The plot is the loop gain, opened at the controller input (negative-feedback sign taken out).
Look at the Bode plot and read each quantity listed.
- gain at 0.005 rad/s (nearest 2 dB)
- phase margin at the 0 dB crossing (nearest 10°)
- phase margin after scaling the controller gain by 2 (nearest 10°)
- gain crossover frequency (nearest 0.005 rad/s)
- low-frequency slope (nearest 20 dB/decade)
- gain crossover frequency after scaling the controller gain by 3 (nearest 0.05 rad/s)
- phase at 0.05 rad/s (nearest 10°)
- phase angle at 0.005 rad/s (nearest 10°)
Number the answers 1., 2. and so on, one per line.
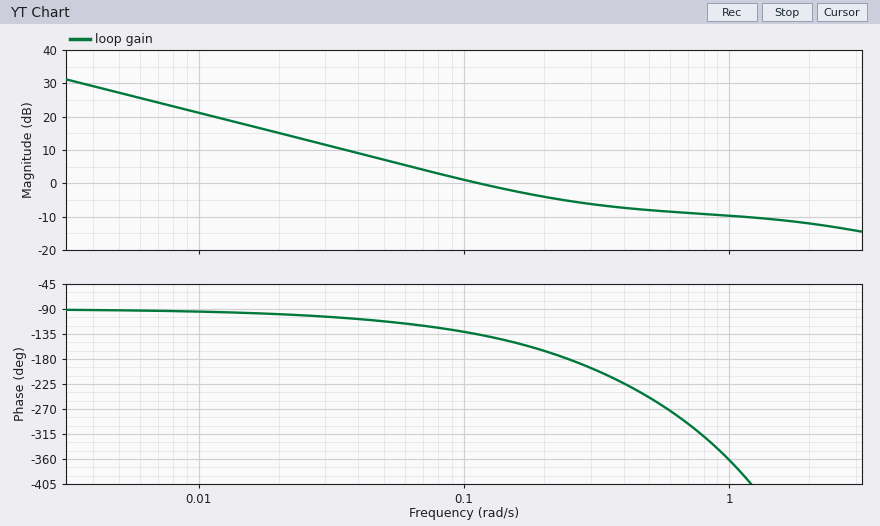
1. 28 dB
2. 40°
3. -10°
4. 0.115 rad/s
5. -20 dB/decade
6. 0.95 rad/s
7. -110°
8. -90°
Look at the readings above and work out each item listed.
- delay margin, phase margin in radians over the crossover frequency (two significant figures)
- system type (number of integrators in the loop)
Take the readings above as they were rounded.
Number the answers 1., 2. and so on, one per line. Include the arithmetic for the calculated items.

1. 40 × π / 180 / 0.115 = 6.1 s
2. 1
